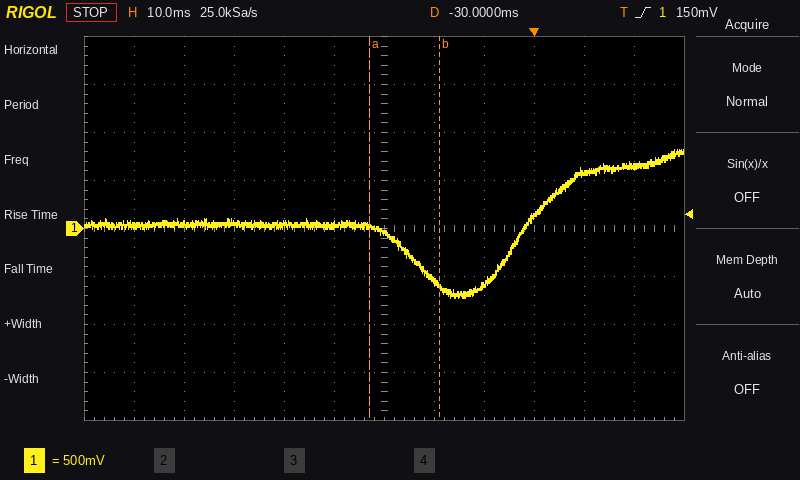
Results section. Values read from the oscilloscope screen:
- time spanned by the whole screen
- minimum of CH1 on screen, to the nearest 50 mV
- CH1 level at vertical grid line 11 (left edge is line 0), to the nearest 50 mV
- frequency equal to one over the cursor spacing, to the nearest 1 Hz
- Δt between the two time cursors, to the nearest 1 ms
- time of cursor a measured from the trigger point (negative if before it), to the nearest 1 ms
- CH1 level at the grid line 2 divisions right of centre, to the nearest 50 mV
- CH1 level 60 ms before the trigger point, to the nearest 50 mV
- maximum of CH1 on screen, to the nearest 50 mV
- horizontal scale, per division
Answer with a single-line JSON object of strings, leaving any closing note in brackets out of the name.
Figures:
{"time spanned by the whole screen": "120 ms", "minimum of CH1 on screen, to the nearest 50 mV": "-700 mV", "CH1 level at vertical grid line 11 (left edge is line 0), to the nearest 50 mV": "650 mV", "frequency equal to one over the cursor spacing, to the nearest 1 Hz": "71 Hz", "Δt between the two time cursors, to the nearest 1 ms": "14 ms", "time of cursor a measured from the trigger point (negative if before it), to the nearest 1 ms": "-33 ms", "CH1 level at the grid line 2 divisions right of centre, to the nearest 50 mV": "-600 mV", "CH1 level 60 ms before the trigger point, to the nearest 50 mV": "50 mV", "maximum of CH1 on screen, to the nearest 50 mV": "800 mV", "horizontal scale, per division": "10 ms"}
